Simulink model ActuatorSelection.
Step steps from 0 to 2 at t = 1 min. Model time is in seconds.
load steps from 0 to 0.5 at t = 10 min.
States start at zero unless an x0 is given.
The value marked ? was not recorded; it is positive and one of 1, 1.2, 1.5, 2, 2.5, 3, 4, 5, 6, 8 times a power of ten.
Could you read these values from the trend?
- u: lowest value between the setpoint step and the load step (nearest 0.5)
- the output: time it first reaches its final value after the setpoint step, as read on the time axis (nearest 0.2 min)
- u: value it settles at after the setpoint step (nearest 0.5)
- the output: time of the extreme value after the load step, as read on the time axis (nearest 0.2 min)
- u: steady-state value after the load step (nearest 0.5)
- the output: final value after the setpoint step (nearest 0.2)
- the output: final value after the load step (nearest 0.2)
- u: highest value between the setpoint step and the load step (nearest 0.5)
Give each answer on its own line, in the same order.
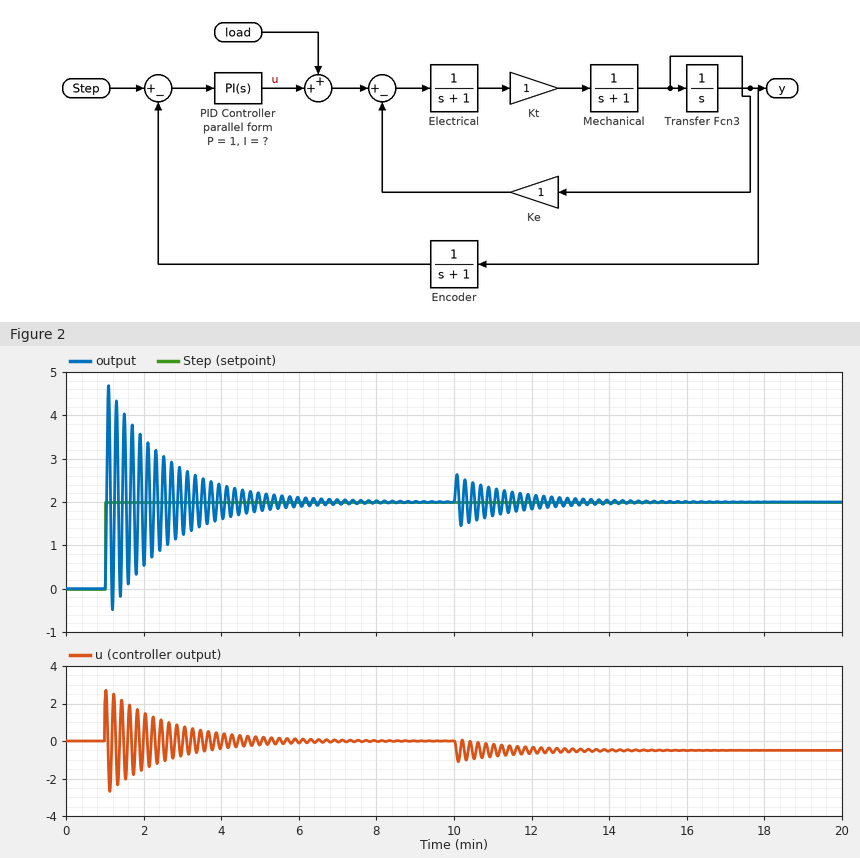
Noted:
-2.5
1.0 min
0.0
10.0 min
-0.5
2.0
2.0
2.5
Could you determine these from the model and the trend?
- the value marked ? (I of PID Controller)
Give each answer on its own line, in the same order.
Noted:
0.3
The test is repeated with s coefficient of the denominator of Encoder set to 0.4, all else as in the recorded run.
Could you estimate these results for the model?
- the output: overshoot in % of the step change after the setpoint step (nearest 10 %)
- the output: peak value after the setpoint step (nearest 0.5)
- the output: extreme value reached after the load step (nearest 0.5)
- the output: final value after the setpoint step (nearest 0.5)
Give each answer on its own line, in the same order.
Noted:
90 %
4.0
2.5
2.0
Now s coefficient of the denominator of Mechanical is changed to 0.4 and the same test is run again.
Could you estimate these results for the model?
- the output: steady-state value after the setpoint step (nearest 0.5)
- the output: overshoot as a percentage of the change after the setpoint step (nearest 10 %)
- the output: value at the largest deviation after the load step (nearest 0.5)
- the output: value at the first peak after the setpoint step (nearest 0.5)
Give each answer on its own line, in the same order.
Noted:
2.0
100 %
2.5
4.0
